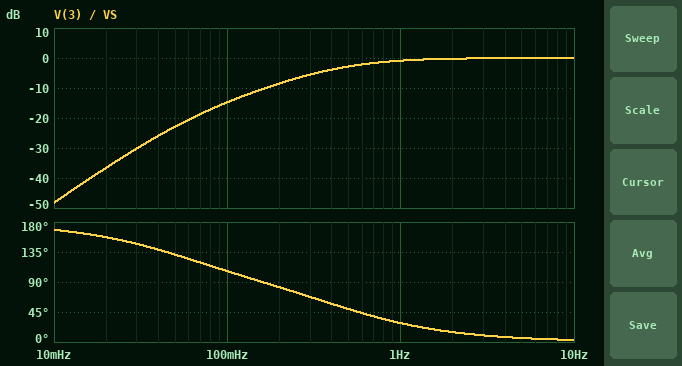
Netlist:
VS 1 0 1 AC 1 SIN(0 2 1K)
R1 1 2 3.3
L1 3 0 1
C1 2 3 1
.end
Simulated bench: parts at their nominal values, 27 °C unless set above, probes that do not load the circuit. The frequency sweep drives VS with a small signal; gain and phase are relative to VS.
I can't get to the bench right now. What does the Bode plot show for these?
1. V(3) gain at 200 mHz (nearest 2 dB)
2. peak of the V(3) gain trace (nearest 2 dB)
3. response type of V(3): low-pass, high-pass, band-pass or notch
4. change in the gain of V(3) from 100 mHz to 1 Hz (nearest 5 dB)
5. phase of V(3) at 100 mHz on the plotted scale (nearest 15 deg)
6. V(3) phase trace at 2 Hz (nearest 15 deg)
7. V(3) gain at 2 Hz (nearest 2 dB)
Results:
-8 dB
0 dB
high-pass
15 dB
105 deg
15 deg
0 dB
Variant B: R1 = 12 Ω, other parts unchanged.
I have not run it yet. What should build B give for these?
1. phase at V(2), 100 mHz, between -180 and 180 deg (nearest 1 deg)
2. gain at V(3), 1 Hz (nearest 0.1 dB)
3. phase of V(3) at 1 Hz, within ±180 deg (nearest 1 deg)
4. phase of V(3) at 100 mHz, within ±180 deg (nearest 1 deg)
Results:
-85 deg
-6.6 dB
63 deg
95 deg
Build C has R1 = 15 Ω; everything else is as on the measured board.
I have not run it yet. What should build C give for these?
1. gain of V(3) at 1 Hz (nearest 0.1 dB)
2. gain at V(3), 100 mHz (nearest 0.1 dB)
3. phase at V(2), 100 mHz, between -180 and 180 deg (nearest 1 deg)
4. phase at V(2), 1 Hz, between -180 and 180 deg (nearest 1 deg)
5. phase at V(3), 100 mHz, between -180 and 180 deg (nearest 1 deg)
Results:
-8.2 dB
-27.6 dB
-86 deg
68 deg
94 deg
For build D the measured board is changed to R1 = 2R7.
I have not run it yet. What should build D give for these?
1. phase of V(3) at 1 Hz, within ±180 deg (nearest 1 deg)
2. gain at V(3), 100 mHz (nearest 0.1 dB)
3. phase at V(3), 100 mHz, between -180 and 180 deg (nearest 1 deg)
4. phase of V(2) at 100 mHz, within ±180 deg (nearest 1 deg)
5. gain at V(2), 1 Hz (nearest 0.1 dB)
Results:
24 deg
-13.2 dB
110 deg
-70 deg
-0.8 dB
